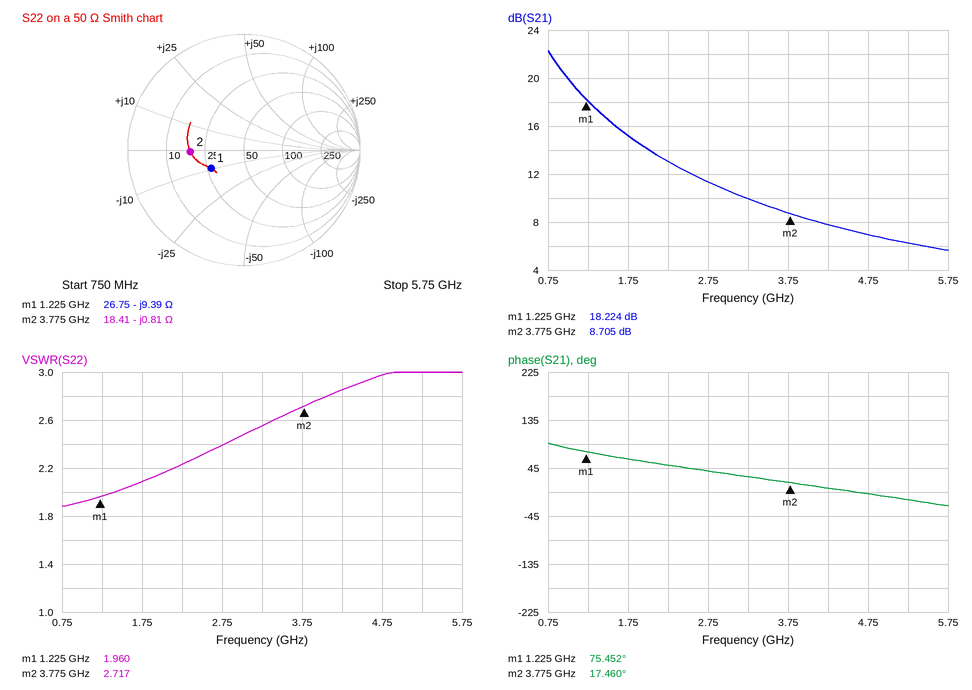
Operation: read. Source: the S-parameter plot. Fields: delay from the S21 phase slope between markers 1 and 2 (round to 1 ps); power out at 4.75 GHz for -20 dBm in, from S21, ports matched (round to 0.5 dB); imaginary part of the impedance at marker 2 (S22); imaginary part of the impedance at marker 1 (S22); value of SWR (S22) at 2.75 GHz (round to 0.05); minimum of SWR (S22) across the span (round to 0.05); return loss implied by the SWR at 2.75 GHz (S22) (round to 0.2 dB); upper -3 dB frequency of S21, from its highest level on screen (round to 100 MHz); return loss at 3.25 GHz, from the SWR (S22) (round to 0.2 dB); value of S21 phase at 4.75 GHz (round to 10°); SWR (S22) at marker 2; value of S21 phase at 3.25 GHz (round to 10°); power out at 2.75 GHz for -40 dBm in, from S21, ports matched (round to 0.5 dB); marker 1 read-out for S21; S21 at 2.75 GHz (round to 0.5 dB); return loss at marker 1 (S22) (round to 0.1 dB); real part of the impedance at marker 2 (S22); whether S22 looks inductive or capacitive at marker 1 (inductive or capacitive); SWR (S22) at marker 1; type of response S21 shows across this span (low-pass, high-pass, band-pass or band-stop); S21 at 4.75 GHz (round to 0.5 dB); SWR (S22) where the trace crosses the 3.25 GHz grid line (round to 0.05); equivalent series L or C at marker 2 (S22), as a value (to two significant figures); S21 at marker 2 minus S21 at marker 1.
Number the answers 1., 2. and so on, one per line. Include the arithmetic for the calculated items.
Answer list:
1. −(17.46° − (75.452°))/(360° × 2.55 GHz) ≈ 63 ps
2. -20 dBm + (7.0 dB) = -13.0 dBm
3. -0.81 Ω
4. -9.39 Ω
5. 2.40
6. 1.90
7. −20 log10((2.4 − 1)/(2.4 + 1)) ≈ 7.71 dB, so 7.8 dB to the nearest 0.2 dB
8. 1.1 GHz
9. −20 log10((2.55 − 1)/(2.55 + 1)) ≈ 7.2 dB
10. 0°
11. 2.717
12. 30°
13. -40 dBm + (11.5 dB) = -28.5 dBm
14. 18.224 dB
15. 11.5 dB
16. 9.8 dB
17. 18.41 Ω
18. capacitive
19. 1.960
20. low-pass
21. 7.0 dB
22. 2.55
23. C = 1/(2π × 3.775 GHz × 0.81 Ω) ≈ 52 pF
24. 8.705 − (18.224) = -9.519 dB
